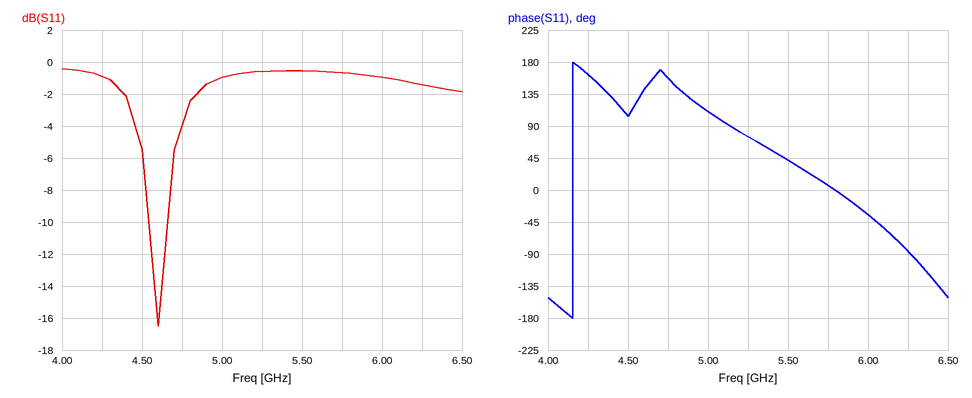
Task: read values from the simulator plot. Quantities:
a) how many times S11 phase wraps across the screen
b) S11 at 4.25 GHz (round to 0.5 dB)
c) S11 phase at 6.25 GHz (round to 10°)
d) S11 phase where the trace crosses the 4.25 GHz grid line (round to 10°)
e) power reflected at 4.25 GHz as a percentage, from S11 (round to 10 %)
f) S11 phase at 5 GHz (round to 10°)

1
-1.0 dB
-90°
160°
80 %
110°
